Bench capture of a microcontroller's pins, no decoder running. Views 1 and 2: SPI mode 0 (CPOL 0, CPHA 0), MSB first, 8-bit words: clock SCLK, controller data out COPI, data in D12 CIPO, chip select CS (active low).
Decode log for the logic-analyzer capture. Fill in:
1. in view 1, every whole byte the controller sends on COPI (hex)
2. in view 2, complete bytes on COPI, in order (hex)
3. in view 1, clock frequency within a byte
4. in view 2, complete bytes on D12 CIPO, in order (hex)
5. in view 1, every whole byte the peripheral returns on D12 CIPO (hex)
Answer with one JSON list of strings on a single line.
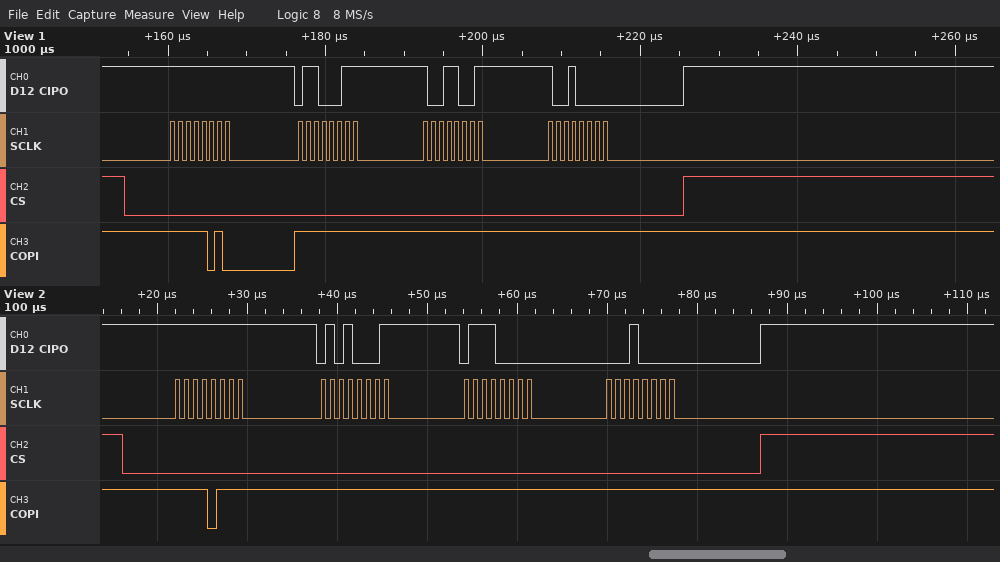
["FA FF FF FF", "F7 FF FF FF", "1 MHz", "FF 51 70 10", "FF 63 99 90"]
